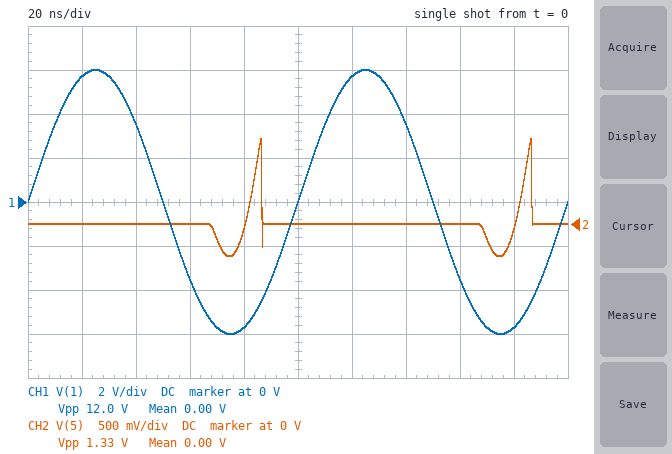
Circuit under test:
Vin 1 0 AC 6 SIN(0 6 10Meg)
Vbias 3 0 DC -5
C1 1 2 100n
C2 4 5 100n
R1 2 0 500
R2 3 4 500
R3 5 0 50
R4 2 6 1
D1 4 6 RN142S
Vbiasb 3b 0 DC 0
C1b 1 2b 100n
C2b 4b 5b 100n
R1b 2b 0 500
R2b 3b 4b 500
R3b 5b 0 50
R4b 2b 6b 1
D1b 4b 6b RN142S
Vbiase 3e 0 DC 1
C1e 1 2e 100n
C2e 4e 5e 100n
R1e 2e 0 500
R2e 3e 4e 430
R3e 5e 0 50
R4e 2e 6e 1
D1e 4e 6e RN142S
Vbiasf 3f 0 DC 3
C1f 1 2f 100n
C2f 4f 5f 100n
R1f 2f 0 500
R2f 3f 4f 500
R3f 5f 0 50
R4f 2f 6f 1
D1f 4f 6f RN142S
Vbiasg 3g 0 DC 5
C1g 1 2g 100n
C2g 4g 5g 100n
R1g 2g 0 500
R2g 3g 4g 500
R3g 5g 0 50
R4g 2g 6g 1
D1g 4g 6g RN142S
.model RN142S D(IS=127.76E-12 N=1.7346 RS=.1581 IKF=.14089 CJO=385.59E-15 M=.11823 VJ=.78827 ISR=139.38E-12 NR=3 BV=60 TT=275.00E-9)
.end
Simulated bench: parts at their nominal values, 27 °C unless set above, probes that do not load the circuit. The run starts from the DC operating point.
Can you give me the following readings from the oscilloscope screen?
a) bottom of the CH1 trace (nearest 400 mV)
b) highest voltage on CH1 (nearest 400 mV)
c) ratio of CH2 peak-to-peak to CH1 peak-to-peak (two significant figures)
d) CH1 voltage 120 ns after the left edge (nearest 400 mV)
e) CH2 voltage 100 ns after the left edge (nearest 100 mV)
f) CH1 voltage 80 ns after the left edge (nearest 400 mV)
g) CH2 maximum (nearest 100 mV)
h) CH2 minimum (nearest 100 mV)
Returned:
-6.0 V
6.0 V
0.11
5.6 V
0 V
-5.6 V
1.0 V
-400 mV
